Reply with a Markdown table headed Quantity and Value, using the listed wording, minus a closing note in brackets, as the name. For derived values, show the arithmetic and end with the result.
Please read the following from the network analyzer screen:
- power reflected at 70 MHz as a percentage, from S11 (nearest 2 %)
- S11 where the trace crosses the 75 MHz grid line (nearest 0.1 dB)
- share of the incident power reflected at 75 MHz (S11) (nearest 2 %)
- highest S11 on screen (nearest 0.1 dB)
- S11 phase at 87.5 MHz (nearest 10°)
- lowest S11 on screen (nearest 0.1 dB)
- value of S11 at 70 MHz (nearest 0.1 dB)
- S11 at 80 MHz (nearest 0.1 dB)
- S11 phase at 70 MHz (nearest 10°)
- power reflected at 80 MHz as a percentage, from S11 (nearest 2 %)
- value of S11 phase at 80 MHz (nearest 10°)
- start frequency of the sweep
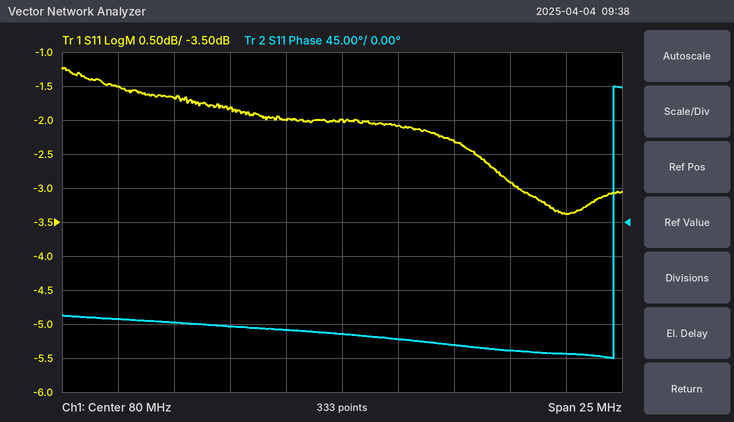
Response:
| Quantity | Value |
|---|---|
| power reflected at 70 MHz as a percentage, from S11 | 10^(-1.5/10) ≈ 70.8 %, so 70 % to the nearest 2 % |
| S11 where the trace crosses the 75 MHz grid line | -1.8 dB |
| share of the incident power reflected at 75 MHz (S11) | 10^(-1.8/10) ≈ 66 % |
| highest S11 on screen | -1.2 dB |
| S11 phase at 87.5 MHz | -170° |
| lowest S11 on screen | -3.4 dB |
| value of S11 at 70 MHz | -1.5 dB |
| S11 at 80 MHz | -2.0 dB |
| S11 phase at 70 MHz | -130° |
| power reflected at 80 MHz as a percentage, from S11 | 10^(-2/10) ≈ 63.1 %, so 64 % to the nearest 2 % |
| value of S11 phase at 80 MHz | -150° |
| start frequency of the sweep | 67.5 MHz |
